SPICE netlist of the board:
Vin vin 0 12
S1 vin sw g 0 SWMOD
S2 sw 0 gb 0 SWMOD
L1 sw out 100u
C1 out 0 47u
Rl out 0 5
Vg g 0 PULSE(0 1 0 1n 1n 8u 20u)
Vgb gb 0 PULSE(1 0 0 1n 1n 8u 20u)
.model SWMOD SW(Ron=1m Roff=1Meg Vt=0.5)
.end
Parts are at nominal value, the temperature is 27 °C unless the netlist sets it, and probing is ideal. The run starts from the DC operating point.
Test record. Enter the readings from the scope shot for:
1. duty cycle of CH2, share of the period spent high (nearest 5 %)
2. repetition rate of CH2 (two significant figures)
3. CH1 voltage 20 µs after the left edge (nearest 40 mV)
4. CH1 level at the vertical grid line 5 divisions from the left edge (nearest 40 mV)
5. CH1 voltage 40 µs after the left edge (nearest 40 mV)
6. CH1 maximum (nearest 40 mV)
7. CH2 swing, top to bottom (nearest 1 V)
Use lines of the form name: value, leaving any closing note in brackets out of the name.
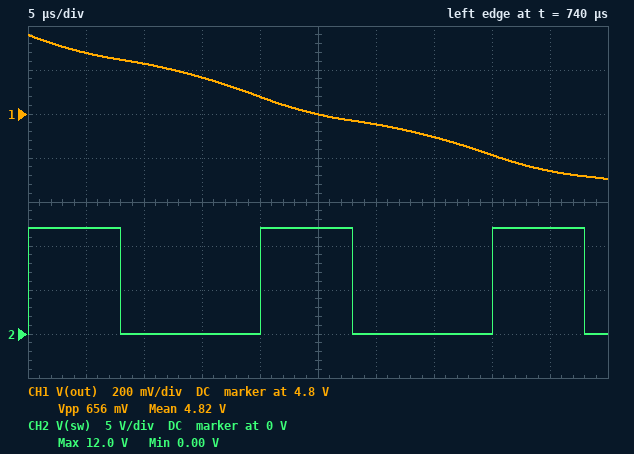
duty cycle of CH2, share of the period spent high: 40 %
repetition rate of CH2: 50 kHz
CH1 voltage 20 µs after the left edge: 4.88 V
CH1 level at the vertical grid line 5 divisions from the left edge: 4.80 V
CH1 voltage 40 µs after the left edge: 4.60 V
CH1 maximum: 5.16 V
CH2 swing, top to bottom: 12 V
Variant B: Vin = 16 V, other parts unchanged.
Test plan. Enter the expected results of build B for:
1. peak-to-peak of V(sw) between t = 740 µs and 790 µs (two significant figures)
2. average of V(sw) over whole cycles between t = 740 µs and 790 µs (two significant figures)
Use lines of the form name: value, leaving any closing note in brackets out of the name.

peak-to-peak of V(sw) between t = 740 µs and 790 µs: 16 V
average of V(sw) over whole cycles between t = 740 µs and 790 µs: 6.4 V
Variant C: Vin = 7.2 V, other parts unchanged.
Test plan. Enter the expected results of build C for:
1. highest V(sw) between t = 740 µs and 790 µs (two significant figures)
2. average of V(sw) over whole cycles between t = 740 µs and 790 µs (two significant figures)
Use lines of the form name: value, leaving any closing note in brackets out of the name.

highest V(sw) between t = 740 µs and 790 µs: 7.2 V
average of V(sw) over whole cycles between t = 740 µs and 790 µs: 2.9 V
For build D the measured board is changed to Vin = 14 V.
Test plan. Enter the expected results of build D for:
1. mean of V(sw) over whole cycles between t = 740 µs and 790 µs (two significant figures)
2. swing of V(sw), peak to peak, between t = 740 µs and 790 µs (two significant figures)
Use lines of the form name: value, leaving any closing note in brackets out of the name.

mean of V(sw) over whole cycles between t = 740 µs and 790 µs: 5.6 V
swing of V(sw), peak to peak, between t = 740 µs and 790 µs: 14 V
